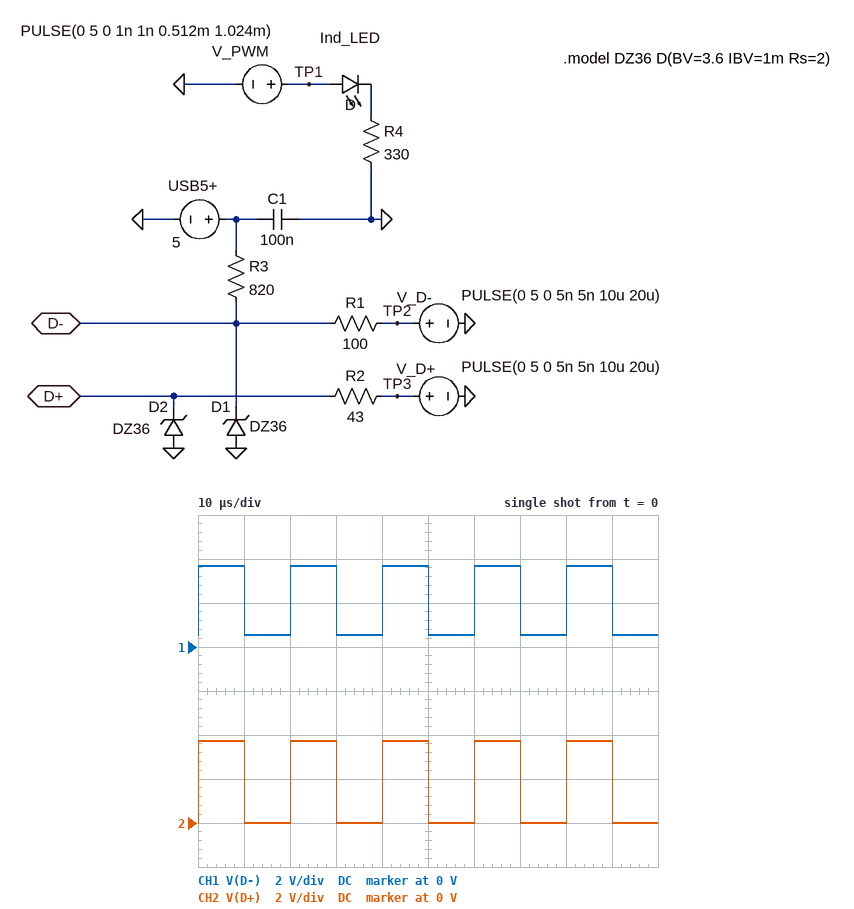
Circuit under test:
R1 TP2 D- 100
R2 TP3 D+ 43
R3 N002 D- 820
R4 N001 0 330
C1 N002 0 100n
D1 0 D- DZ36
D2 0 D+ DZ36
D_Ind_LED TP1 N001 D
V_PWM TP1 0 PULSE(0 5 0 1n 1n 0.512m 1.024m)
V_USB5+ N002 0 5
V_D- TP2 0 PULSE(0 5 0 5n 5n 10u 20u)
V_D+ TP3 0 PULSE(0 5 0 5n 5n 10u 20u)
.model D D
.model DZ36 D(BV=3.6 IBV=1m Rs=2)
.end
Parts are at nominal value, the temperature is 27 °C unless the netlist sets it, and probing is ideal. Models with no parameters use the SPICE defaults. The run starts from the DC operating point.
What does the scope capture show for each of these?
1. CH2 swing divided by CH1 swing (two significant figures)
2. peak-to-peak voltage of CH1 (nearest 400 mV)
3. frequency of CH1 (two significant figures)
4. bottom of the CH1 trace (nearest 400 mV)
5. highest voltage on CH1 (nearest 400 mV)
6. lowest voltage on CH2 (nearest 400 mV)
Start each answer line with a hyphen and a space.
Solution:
- 1.2
- 3.2 V
- 50 kHz
- 400 mV
- 3.6 V
- 0 V
